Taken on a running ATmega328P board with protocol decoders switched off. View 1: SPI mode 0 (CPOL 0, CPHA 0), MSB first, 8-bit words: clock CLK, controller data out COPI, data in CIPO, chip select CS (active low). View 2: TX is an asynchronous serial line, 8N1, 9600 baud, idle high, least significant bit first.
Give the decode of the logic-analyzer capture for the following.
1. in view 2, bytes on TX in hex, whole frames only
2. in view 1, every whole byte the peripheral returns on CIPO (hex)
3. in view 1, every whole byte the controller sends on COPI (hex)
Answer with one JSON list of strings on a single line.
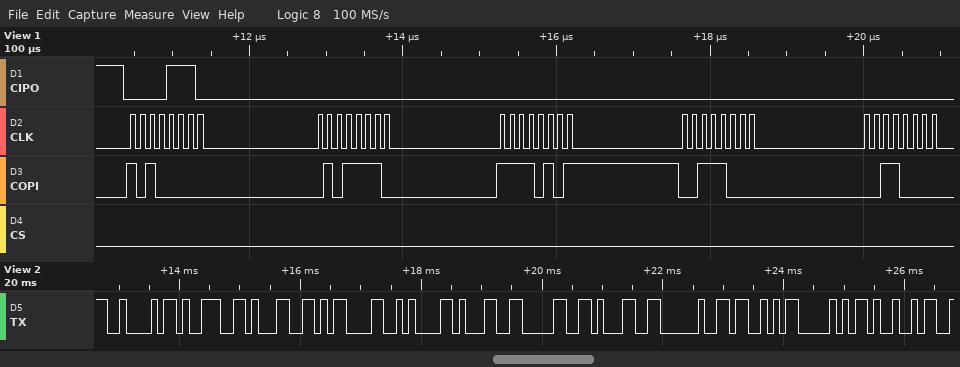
["0x42 0x39 0x31 0x0D 0x0A 0x31 0x30 0x31 0x20 0x53 0x50 0x49", "0E 00 00 00 00", "A0 5E F5 38 30"]
